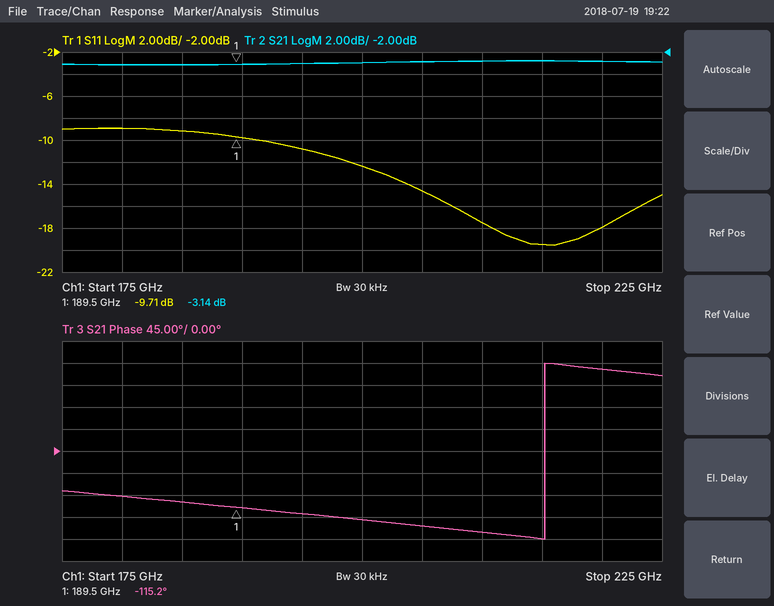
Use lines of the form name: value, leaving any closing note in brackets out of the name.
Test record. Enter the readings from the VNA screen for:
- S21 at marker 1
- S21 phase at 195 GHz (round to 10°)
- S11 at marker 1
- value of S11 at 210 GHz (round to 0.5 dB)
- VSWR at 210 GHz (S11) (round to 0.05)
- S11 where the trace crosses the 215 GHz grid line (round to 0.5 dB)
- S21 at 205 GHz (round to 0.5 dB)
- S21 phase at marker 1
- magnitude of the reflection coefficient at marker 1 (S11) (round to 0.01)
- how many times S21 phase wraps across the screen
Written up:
S21 at marker 1: -3.14 dB
S21 phase at 195 GHz: -130°
S11 at marker 1: -9.71 dB
value of S11 at 210 GHz: -17.5 dB
VSWR at 210 GHz (S11): 1.30
S11 where the trace crosses the 215 GHz grid line: -19.5 dB
S21 at 205 GHz: -3.0 dB
S21 phase at marker 1: -115.2°
magnitude of the reflection coefficient at marker 1 (S11): 0.33
how many times S21 phase wraps across the screen: 1
